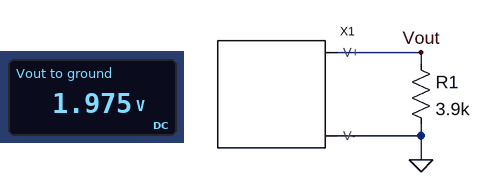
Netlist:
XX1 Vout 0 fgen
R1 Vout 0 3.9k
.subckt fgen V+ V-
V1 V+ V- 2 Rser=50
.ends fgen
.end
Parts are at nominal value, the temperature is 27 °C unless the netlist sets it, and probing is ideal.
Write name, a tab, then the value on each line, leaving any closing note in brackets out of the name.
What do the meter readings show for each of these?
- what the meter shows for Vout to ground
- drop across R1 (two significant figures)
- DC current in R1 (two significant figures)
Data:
what the meter shows for Vout to ground	1.975 V
drop across R1	2.0 V
DC current in R1	510 µA
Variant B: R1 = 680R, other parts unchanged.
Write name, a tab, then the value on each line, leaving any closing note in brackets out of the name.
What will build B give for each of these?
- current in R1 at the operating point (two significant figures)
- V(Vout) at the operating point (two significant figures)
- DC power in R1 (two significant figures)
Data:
current in R1 at the operating point	2.7 mA
V(Vout) at the operating point	1.9 V
DC power in R1	5.1 mW
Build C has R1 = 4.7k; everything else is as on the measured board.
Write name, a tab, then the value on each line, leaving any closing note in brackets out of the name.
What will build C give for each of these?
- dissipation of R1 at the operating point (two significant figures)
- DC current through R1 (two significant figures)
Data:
dissipation of R1 at the operating point	830 µW
DC current through R1	420 µA
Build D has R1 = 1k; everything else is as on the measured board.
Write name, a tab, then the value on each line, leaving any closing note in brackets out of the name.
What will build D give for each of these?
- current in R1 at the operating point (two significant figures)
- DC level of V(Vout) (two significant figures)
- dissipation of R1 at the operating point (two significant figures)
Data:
current in R1 at the operating point	1.9 mA
DC level of V(Vout)	1.9 V
dissipation of R1 at the operating point	3.6 mW
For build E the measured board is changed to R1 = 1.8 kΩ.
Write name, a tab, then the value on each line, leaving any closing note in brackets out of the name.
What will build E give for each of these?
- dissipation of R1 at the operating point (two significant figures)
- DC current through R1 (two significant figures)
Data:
dissipation of R1 at the operating point	2.1 mW
DC current through R1	1.1 mA
